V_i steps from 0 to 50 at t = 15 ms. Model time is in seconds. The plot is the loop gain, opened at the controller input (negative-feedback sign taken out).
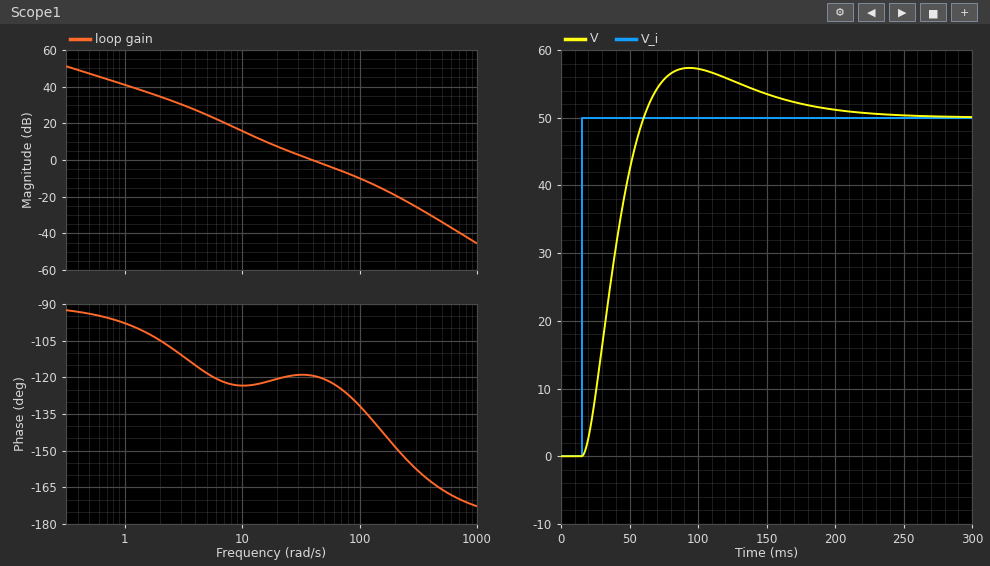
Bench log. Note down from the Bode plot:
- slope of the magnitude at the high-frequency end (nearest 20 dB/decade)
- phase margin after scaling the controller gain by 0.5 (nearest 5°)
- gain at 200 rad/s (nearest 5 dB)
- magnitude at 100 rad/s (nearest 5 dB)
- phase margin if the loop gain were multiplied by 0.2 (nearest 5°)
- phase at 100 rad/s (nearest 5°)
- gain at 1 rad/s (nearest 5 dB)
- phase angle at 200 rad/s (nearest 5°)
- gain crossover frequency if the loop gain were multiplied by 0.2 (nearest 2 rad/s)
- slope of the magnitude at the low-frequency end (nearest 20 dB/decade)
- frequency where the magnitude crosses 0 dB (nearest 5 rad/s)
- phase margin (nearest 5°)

-40 dB/decade
60°
-20 dB
-10 dB
55°
-130°
40 dB
-150°
12 rad/s
-20 dB/decade
40 rad/s
60°
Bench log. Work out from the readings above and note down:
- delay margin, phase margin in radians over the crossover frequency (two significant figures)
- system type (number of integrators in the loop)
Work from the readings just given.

0.026 s
1
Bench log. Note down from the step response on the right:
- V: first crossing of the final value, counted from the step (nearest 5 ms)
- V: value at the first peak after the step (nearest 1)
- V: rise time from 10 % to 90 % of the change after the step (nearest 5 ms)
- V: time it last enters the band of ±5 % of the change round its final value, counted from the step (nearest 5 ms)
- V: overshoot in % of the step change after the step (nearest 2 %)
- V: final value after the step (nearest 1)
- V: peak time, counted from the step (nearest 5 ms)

45 ms
57
30 ms
150 ms
14 %
50
80 ms
